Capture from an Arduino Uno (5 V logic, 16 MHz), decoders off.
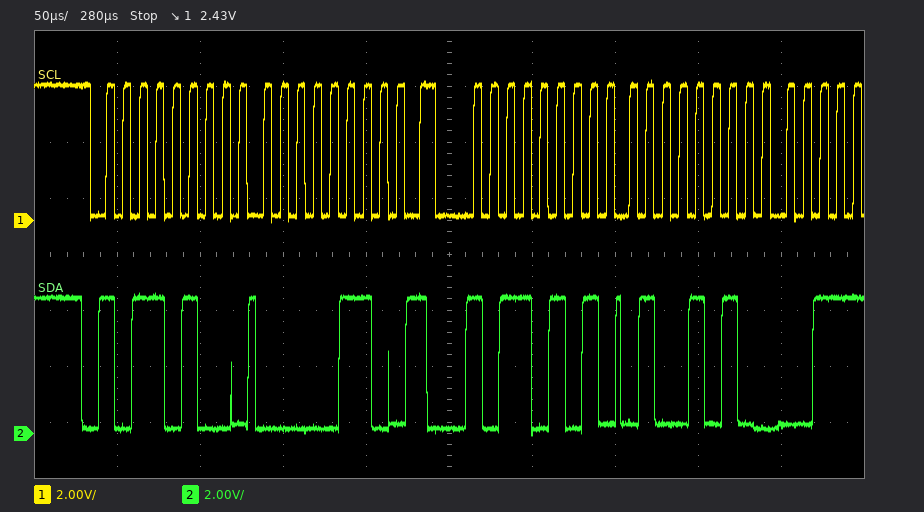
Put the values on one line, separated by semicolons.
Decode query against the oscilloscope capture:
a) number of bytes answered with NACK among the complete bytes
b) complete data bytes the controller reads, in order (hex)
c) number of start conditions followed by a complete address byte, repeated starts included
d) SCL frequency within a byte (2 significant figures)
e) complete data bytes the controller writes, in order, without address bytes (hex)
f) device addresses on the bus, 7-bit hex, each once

0; 4A; 2; 100 kHz; 06; 0x5A
